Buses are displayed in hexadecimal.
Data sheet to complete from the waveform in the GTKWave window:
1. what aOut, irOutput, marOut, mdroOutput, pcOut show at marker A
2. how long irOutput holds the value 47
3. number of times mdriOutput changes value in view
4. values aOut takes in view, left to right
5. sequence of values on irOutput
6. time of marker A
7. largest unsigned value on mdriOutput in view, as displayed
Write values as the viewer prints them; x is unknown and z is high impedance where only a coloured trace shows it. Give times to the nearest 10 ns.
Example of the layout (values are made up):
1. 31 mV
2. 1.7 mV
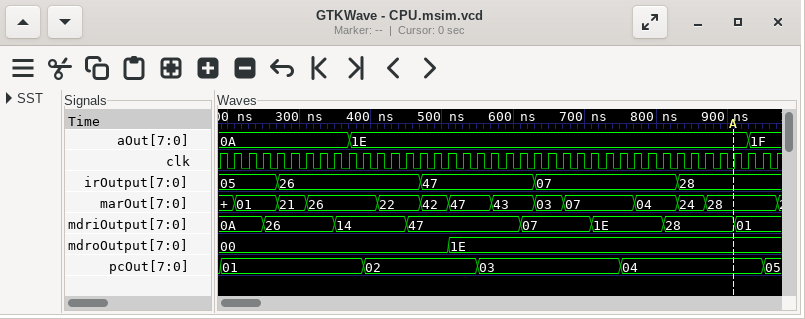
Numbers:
1. aOut=1E, irOutput=28, marOut=28, mdroOutput=1E, pcOut=04
2. 160 ns
3. 7
4. 0A, 1E, 1F
5. 05, 26, 47, 07, 28
6. 910 ns
7. 47
